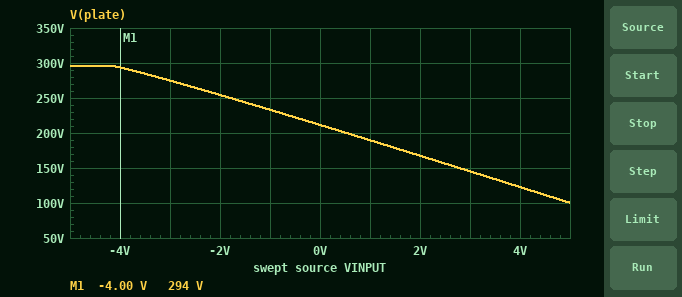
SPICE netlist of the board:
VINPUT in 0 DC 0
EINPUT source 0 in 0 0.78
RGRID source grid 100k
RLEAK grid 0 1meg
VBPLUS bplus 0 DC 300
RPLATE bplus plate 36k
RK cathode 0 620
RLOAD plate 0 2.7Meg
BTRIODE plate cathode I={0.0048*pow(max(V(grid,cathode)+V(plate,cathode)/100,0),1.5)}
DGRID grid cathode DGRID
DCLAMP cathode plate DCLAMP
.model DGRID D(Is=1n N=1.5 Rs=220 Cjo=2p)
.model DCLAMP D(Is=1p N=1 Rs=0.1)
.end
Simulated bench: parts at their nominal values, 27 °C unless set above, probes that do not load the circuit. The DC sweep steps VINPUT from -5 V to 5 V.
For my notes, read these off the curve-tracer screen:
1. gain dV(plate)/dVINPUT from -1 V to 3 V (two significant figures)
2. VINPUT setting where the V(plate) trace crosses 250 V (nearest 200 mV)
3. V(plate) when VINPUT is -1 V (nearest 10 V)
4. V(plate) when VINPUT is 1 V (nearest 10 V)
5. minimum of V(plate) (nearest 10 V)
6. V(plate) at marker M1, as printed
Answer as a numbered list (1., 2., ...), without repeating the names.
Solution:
1. -22 V/V
2. -1.8 V
3. 230 V
4. 190 V
5. 100 V
6. 294 V
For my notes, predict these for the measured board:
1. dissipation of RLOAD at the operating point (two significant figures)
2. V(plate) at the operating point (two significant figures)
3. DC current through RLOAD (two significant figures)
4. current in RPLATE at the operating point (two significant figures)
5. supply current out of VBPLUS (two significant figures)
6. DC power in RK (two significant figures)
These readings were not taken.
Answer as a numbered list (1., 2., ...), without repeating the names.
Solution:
1. 17 mW
2. 210 V
3. 78 µA
4. 2.5 mA
5. 2.5 mA
6. 3.5 mW
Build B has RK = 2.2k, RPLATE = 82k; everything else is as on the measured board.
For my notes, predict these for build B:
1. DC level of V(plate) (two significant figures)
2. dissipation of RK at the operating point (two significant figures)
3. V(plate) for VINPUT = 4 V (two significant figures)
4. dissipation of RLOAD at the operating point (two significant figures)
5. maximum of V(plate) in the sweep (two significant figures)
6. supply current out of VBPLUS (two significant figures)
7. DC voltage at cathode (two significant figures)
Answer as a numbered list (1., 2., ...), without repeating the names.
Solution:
1. 220 V
2. 1.6 mW
3. 150 V
4. 18 mW
5. 290 V
6. 940 µA
7. 1.9 V
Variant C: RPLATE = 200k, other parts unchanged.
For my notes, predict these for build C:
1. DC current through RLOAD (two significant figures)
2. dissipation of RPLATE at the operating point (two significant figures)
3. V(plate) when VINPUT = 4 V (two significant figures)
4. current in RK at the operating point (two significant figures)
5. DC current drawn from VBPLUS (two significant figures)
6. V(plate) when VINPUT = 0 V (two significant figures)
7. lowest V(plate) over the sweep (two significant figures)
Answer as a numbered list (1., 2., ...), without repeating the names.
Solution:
1. 36 µA
2. 210 mW
3. 7.9 V
4. 980 µA
5. 1.0 mA
6. 96 V
7. 6.5 V
